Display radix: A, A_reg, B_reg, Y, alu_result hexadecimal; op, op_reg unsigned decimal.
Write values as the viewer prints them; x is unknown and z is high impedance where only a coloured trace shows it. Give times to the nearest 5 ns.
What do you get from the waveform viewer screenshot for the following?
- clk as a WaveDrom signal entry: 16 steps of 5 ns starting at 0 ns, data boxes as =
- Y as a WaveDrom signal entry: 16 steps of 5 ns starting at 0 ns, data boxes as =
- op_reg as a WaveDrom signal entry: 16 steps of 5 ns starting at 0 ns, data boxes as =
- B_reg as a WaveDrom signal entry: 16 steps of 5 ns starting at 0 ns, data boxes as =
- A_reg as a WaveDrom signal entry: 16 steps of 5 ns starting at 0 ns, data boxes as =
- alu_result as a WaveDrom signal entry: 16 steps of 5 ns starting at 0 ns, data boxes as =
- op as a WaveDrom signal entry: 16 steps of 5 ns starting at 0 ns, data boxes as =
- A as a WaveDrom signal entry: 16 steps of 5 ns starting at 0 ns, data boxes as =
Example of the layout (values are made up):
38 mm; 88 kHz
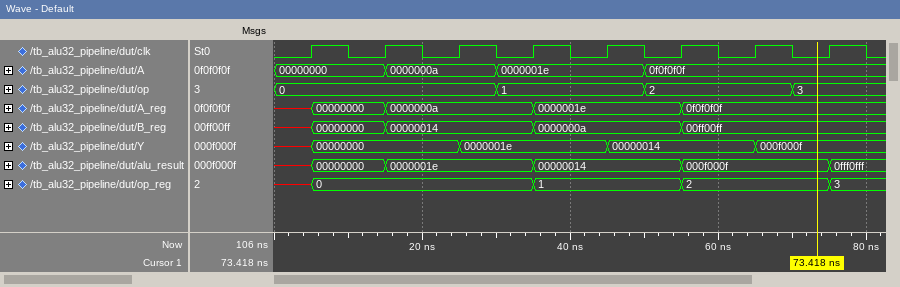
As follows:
{name: 'clk', wave: '0101010101010101'}; {name: 'Y', wave: 'x=...=...=...=..', data: '00000000 0000001e 00000014 000f000f'}; {name: 'op_reg', wave: 'x=.....=...=...=', data: '0 1 2 3'}; {name: 'B_reg', wave: 'x=.=...=...=....', data: '00000000 00000014 0000000a 00ff00ff'}; {name: 'A_reg', wave: 'x=.=...=...=....', data: '00000000 0000000a 0000001e 0f0f0f0f'}; {name: 'alu_result', wave: 'x=.=...=...=...=', data: '00000000 0000001e 00000014 000f000f 0fff0fff'}; {name: 'op', wave: '=.....=...=...=.', data: '0 1 2 3'}; {name: 'A', wave: '=..=..=...=.....', data: '00000000 0000000a 0000001e 0f0f0f0f'}
